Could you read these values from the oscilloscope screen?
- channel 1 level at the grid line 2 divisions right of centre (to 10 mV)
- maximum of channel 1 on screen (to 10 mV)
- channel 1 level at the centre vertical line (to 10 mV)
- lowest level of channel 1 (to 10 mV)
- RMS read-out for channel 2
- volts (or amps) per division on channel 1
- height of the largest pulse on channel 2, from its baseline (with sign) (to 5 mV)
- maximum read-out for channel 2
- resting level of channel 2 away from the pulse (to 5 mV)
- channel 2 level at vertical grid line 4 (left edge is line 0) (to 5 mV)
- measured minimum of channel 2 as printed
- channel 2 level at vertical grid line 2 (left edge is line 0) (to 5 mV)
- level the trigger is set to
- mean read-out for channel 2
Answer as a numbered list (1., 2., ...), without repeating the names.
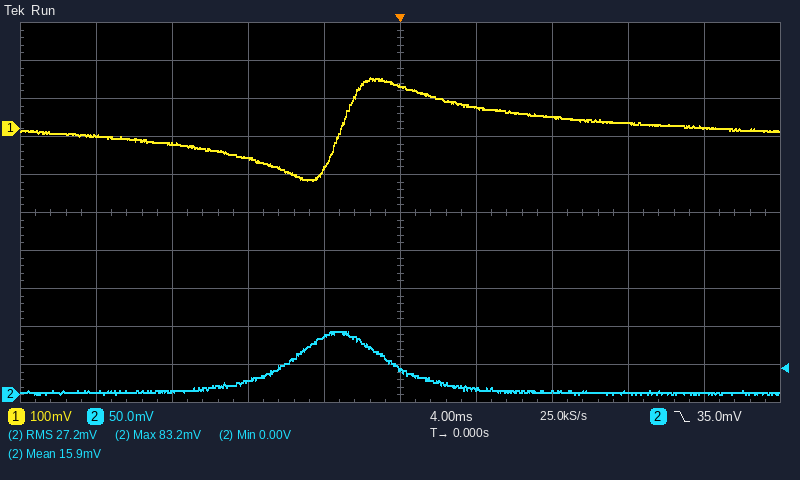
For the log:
1. 30 mV
2. 140 mV
3. 110 mV
4. -140 mV
5. 27.2 mV
6. 100 mV
7. +80 mV
8. 83.2 mV
9. 5 mV
10. 75 mV
11. 0.00 V
12. 5 mV
13. 35.0 mV
14. 15.9 mV
